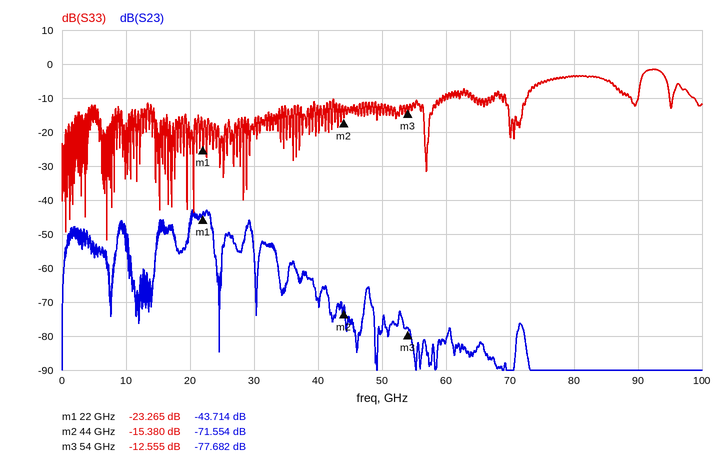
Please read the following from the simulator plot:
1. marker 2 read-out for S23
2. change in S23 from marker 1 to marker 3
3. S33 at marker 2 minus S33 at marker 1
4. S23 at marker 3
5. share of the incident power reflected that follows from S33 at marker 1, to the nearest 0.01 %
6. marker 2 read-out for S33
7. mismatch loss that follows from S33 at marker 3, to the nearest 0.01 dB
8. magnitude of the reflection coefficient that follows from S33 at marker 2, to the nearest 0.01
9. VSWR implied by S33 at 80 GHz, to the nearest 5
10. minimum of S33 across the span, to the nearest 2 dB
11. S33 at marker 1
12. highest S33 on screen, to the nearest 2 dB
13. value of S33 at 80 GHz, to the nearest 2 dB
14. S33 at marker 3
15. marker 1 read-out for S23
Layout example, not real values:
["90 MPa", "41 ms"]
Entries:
["-71.554 dB", "-33.968 dB", "7.885 dB", "-77.682 dB", "0.47 %", "-15.380 dB", "0.25 dB", "0.17", "5", "-52 dB", "-23.265 dB", "-2 dB", "-4 dB", "-12.555 dB", "-43.714 dB"]
